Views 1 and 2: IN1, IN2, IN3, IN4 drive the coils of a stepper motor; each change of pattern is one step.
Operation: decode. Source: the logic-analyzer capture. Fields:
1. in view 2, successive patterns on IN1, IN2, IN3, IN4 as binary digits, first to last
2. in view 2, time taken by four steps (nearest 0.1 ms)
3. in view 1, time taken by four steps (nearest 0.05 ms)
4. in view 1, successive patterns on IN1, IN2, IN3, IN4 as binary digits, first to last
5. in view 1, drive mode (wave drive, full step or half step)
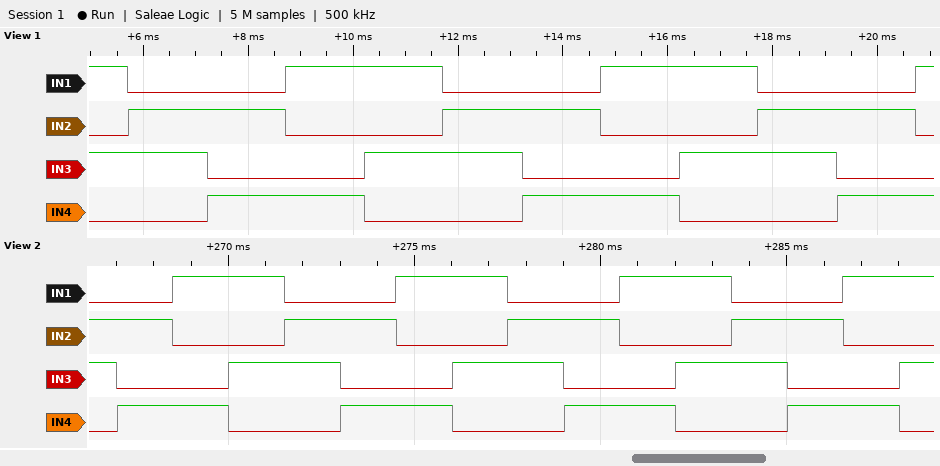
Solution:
0110 0101 1001 1010 0110 0101 1001 1010 0110 0101 1001 1010 0110 0101 1001 1010
6.0 ms
6.00 ms
1010 0110 0101 1001 1010 0110 0101 1001 1010 0110 0101 1001
full step
